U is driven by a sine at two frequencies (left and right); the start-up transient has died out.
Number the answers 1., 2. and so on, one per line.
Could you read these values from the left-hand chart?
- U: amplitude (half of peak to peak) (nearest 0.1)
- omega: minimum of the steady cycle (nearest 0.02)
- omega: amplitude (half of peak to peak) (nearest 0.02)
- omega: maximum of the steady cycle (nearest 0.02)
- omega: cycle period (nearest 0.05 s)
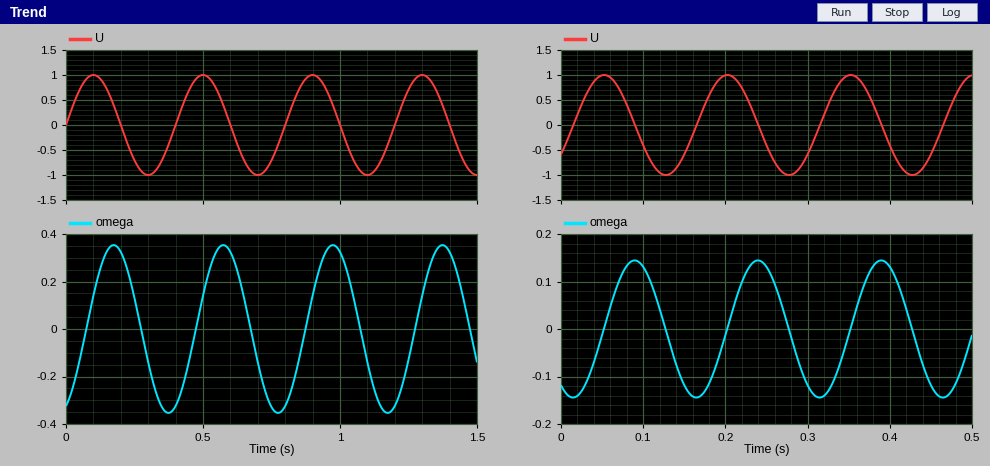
1. 1.0
2. -0.36
3. 0.36
4. 0.36
5. 0.40 s
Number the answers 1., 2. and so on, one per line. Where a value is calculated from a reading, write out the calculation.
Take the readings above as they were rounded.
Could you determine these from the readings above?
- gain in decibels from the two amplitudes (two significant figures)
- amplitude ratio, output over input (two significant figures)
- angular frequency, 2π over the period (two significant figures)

1. 20 log10(0.36 / 1) = -8.9 dB
2. 0.36 / 1 = 0.36
3. 2π / 0.4 = 16 rad/s
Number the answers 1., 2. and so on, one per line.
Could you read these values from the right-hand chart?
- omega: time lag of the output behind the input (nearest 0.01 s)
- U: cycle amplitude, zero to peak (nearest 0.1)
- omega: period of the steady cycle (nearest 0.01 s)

1. 0.04 s
2. 1.0
3. 0.15 s
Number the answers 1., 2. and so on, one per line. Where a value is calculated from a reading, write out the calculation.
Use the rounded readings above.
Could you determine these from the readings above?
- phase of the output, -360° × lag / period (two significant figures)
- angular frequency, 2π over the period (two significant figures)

1. -360 × 0.04 / 0.15 = -96°
2. 2π / 0.15 = 42 rad/s
